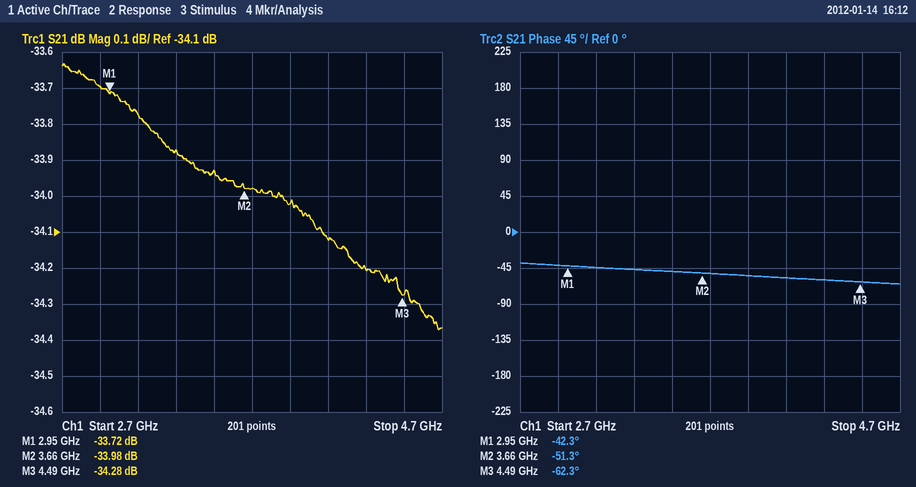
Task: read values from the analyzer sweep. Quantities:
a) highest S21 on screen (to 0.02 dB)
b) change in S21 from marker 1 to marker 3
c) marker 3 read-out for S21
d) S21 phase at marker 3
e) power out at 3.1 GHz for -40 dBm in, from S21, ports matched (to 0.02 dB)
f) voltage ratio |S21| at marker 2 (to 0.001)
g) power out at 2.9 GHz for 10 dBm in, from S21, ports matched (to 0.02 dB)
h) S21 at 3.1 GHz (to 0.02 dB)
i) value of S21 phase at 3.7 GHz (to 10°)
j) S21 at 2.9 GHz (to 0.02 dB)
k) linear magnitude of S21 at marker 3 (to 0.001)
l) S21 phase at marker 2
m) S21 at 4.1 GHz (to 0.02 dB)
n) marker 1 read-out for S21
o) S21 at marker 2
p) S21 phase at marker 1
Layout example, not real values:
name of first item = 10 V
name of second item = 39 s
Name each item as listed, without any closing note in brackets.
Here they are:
highest S21 on screen = -33.64 dB
change in S21 from marker 1 to marker 3 = -0.56 dB
marker 3 read-out for S21 = -34.28 dB
S21 phase at marker 3 = -62.3°
power out at 3.1 GHz for -40 dBm in, from S21, ports matched = -73.78 dBm
voltage ratio |S21| at marker 2 = 0.020
power out at 2.9 GHz for 10 dBm in, from S21, ports matched = -23.70 dBm
S21 at 3.1 GHz = -33.78 dB
value of S21 phase at 3.7 GHz = -50°
S21 at 2.9 GHz = -33.70 dB
linear magnitude of S21 at marker 3 = 0.019
S21 phase at marker 2 = -51.3°
S21 at 4.1 GHz = -34.12 dB
marker 1 read-out for S21 = -33.72 dB
S21 at marker 2 = -33.98 dB
S21 phase at marker 1 = -42.3°
